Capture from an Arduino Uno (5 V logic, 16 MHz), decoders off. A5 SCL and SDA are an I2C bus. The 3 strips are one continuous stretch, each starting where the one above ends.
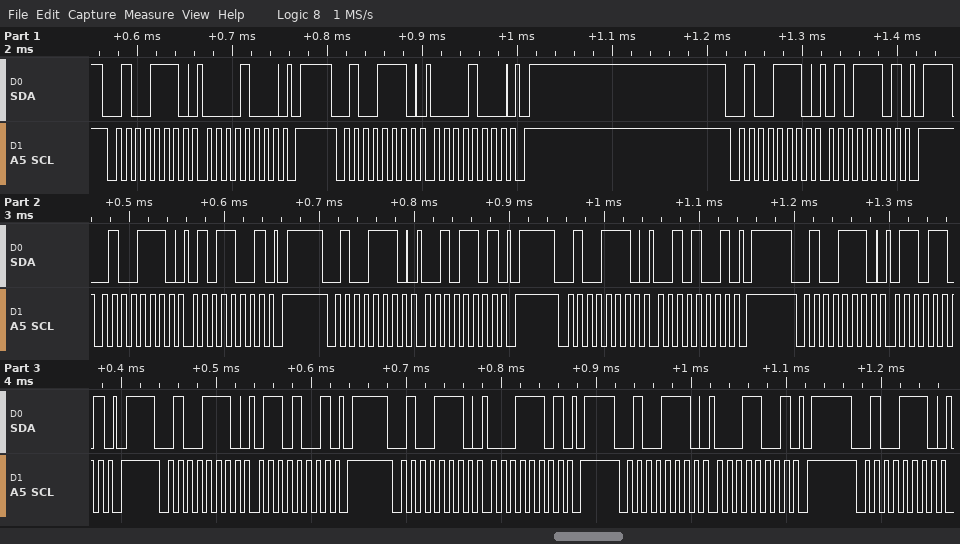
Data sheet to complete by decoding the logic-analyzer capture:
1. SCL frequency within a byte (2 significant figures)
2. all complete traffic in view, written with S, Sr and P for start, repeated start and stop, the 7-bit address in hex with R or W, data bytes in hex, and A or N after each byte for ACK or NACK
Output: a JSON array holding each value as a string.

["100 kHz", "S 27W A 08 A P S 27W A 08 A P S 27W A 5D A P S 27W A 59 A P S 27W A 2D A P S 27W A 29 A P S 27W A 6D A P S 27W A 69 A P S 27W A 1D A P S 27W A 19 A P S 27W A"]
